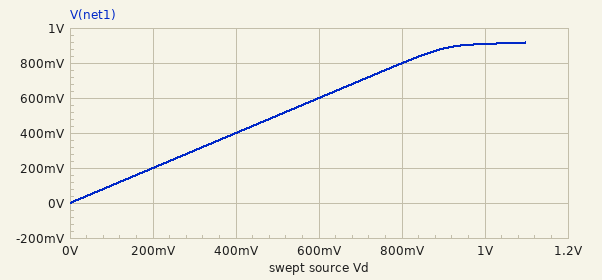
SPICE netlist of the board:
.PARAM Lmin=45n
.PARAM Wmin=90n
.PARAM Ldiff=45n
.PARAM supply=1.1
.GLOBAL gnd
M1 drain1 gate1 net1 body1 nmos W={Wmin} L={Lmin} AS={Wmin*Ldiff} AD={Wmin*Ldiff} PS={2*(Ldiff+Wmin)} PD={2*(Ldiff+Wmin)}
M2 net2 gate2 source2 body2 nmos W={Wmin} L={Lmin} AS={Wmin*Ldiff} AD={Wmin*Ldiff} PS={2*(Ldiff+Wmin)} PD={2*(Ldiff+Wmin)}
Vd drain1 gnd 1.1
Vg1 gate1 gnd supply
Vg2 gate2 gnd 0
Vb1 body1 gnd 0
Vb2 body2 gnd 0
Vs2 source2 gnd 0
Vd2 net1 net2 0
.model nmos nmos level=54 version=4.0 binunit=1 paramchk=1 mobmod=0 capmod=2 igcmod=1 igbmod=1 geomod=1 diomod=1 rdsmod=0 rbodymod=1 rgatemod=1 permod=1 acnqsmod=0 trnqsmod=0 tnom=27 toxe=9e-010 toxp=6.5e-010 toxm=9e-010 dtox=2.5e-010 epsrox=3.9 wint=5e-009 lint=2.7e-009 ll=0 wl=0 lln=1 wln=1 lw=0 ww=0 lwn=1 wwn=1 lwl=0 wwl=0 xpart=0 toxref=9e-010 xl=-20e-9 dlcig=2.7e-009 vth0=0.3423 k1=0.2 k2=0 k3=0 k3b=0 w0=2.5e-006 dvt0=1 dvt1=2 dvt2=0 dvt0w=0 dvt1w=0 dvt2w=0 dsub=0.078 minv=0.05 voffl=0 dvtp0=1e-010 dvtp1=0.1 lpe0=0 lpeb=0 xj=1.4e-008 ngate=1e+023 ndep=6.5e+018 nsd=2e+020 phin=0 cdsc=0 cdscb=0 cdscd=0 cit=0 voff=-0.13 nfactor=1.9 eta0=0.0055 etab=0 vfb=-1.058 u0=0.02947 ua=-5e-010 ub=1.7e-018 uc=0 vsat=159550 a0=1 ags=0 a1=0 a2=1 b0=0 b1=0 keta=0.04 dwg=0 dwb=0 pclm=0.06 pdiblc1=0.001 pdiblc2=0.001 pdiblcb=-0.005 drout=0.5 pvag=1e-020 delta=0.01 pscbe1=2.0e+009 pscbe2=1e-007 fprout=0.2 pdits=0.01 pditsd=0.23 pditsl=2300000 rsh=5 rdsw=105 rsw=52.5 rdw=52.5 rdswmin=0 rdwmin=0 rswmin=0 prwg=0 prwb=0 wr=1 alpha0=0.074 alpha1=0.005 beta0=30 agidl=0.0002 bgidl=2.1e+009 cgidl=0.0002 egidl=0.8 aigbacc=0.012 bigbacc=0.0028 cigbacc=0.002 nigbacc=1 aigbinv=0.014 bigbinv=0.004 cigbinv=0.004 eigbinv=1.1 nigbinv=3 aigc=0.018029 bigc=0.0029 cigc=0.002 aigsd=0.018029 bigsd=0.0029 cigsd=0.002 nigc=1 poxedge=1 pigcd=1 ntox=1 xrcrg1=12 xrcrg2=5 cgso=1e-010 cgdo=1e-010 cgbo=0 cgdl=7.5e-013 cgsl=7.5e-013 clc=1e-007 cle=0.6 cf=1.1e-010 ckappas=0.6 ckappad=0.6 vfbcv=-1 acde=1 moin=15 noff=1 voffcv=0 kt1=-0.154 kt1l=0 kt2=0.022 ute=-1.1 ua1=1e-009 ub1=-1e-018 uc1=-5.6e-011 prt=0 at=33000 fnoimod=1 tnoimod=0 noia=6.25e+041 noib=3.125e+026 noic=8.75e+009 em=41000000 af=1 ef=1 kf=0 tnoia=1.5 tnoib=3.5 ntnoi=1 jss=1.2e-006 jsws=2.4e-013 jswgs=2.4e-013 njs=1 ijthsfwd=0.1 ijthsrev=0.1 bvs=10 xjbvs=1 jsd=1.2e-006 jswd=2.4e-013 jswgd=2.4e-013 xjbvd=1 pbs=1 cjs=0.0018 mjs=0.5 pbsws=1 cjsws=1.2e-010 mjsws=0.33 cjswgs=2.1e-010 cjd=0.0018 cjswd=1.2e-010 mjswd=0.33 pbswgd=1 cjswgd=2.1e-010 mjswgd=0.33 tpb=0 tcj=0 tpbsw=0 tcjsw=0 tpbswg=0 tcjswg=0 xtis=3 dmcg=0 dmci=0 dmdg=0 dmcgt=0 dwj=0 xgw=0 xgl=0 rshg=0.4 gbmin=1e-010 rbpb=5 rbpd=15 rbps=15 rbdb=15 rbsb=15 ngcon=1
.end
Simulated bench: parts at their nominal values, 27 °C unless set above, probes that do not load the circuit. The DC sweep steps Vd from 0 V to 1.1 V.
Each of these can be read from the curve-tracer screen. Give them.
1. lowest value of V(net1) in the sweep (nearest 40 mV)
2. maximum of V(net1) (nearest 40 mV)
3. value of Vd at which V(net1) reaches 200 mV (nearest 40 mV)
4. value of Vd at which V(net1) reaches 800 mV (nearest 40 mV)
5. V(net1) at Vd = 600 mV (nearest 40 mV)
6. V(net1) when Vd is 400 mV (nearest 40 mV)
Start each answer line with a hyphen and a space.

- 0 V
- 920 mV
- 200 mV
- 800 mV
- 600 mV
- 400 mV
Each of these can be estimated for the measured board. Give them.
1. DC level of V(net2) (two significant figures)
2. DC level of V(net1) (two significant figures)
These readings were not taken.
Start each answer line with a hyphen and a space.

- 920 mV
- 920 mV
